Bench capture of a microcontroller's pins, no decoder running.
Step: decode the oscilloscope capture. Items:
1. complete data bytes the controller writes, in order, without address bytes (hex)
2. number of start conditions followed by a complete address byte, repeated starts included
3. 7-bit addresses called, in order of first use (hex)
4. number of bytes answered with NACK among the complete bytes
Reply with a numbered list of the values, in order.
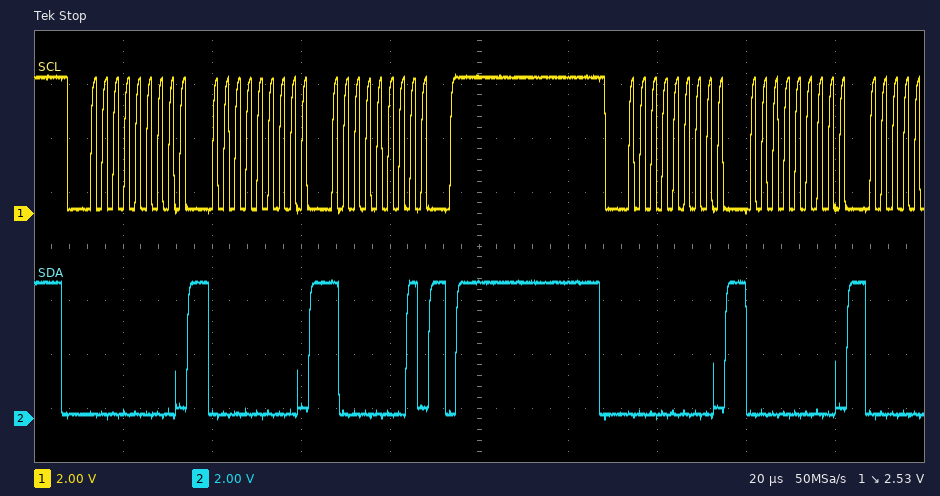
1. 00 81 00
2. 2
3. 0x00
4. 0
